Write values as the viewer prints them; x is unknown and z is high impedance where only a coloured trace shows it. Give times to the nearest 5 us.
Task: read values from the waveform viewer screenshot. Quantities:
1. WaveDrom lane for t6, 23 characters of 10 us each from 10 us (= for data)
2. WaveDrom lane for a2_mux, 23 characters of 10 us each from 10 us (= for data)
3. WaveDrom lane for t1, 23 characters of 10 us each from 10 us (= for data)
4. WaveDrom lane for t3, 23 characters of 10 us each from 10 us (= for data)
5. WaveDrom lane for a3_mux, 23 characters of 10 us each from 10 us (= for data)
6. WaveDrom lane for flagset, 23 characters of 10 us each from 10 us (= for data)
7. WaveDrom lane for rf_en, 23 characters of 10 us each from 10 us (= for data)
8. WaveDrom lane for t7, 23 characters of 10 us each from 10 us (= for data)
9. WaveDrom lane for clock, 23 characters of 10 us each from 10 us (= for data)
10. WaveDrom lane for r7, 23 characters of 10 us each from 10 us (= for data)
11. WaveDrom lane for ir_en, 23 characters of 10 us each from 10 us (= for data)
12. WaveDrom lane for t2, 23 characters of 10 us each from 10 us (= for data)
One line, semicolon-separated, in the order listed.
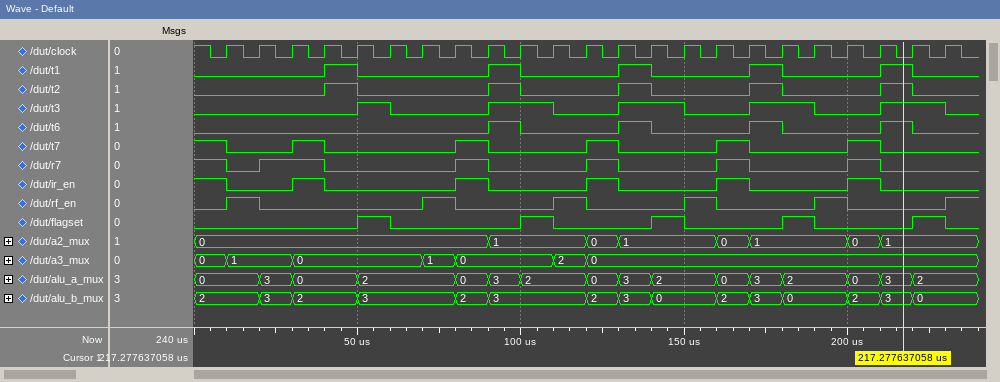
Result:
{name: 't6', wave: '0.......10..10..10..10.'}; {name: 'a2_mux', wave: '=.......=..==..==..==..', data: '0 1 0 1 0 1 0 1'}; {name: 't1', wave: '0..10...10..10..10..10.'}; {name: 't3', wave: '0...10..1.0.1.0.1.0.1.0'}; {name: 'a3_mux', wave: '=.=...==..==...........', data: '1 0 1 0 2 0'}; {name: 'flagset', wave: '0...10...10..10..10..10'}; {name: 'rf_en', wave: '10....10..10..10..10..1'}; {name: 't7', wave: '0.10...10..10..10..10..'}; {name: 'clock', wave: 'p......................'}; {name: 'r7', wave: '01.0...10..10..10..10..'}; {name: 'ir_en', wave: '0.10...10..10..10..10..'}; {name: 't2', wave: '0..10...10..10..10..10.'}
